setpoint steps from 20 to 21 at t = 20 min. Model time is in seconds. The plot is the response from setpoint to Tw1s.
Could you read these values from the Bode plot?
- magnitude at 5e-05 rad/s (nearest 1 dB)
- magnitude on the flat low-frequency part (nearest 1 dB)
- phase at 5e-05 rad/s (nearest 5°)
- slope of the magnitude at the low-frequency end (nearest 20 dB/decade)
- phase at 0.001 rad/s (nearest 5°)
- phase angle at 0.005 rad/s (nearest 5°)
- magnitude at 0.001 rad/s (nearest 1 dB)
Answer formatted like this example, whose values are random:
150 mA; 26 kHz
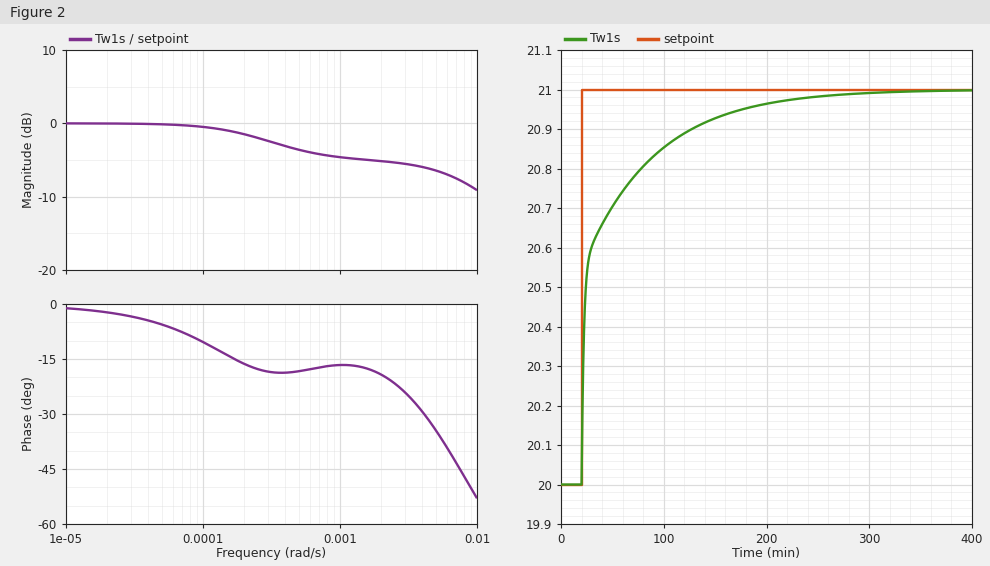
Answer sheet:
0 dB; 0 dB; -5°; 0 dB/decade; -15°; -35°; -5 dB
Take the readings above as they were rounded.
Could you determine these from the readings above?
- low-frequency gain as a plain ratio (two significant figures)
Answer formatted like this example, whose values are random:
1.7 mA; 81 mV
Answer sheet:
1.0
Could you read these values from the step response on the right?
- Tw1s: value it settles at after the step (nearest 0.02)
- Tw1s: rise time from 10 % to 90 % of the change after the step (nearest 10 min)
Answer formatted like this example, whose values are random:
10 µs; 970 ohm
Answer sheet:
21.00; 110 min
